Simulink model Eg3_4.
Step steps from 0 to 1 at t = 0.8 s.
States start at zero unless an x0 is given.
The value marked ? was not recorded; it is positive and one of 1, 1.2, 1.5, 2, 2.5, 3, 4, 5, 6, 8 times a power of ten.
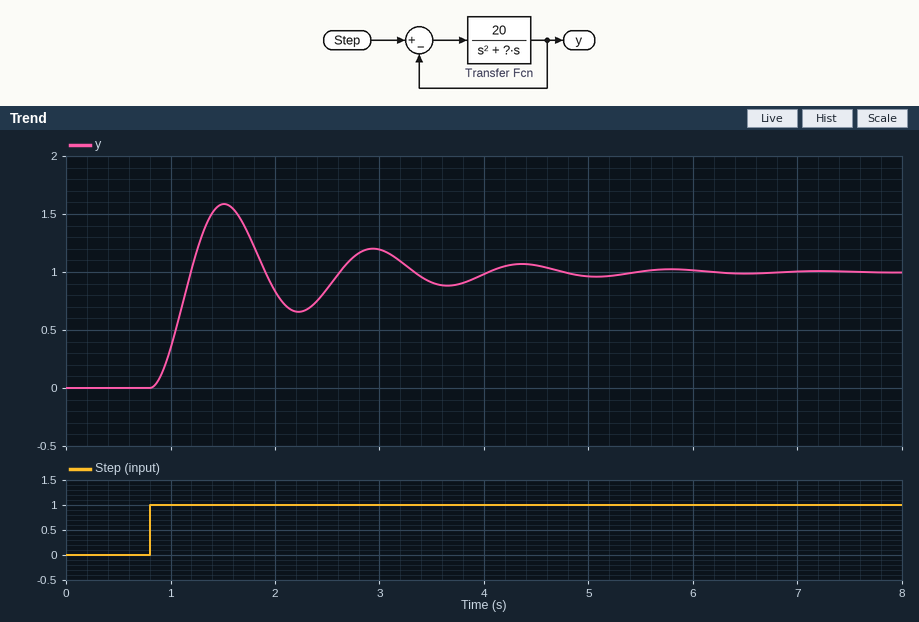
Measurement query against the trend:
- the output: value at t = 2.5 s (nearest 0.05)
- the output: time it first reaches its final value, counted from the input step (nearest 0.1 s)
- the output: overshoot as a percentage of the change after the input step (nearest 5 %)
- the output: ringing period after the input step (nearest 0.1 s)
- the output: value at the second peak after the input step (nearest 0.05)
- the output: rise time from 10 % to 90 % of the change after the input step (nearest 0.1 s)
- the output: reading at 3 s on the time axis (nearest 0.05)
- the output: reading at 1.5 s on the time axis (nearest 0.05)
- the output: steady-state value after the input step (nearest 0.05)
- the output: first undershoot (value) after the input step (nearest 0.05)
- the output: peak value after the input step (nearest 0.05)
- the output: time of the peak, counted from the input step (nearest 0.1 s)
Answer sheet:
0.85
0.4 s
60 %
1.4 s
1.20
0.3 s
1.20
1.60
1.00
0.65
1.60
0.7 s
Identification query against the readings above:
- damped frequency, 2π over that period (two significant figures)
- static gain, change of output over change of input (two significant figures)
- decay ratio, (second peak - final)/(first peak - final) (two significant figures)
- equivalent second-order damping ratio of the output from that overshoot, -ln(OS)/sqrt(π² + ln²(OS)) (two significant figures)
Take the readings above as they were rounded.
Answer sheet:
4.5 rad/s
1.0
0.33
0.16
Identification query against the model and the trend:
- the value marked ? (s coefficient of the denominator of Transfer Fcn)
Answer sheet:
1.5
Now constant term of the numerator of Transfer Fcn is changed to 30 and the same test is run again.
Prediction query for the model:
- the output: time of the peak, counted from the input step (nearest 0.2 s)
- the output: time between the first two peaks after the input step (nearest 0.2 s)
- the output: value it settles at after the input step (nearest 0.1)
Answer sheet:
0.6 s
1.2 s
1.0
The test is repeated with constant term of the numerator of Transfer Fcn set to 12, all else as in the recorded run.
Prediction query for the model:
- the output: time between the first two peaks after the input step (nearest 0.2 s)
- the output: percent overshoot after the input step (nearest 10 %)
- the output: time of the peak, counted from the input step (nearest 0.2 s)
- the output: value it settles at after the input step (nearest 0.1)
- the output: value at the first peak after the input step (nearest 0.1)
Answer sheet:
1.8 s
50 %
1.0 s
1.0
1.5
